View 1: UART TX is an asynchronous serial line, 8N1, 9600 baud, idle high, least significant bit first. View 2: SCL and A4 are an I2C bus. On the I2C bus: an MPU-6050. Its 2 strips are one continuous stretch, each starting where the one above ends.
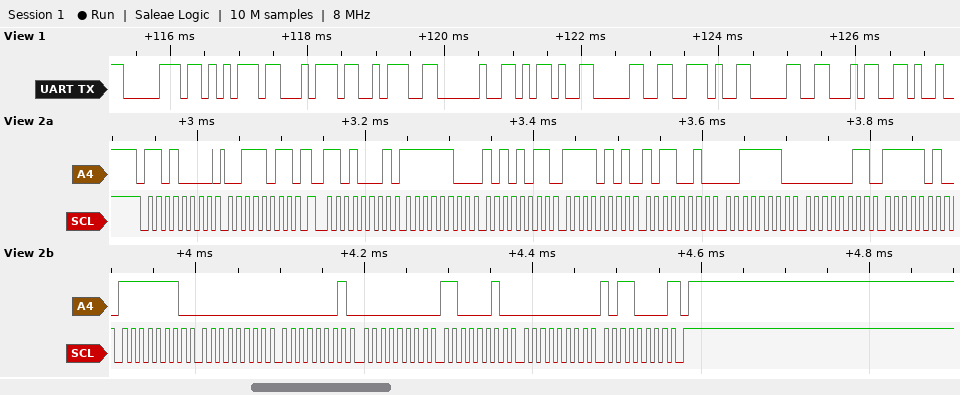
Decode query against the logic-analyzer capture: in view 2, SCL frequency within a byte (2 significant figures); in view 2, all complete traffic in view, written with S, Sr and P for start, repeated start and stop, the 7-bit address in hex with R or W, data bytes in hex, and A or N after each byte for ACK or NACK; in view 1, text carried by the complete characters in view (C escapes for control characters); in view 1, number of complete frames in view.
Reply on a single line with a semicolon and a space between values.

100 kHz; S 68W A 3B A Sr 68R A FC A AB A F5 A B2 A 3E A 03 A FA A FE A 00 A 01 A 00 A C2 A 00 A B0 N P; "put: -0.04"; 10
